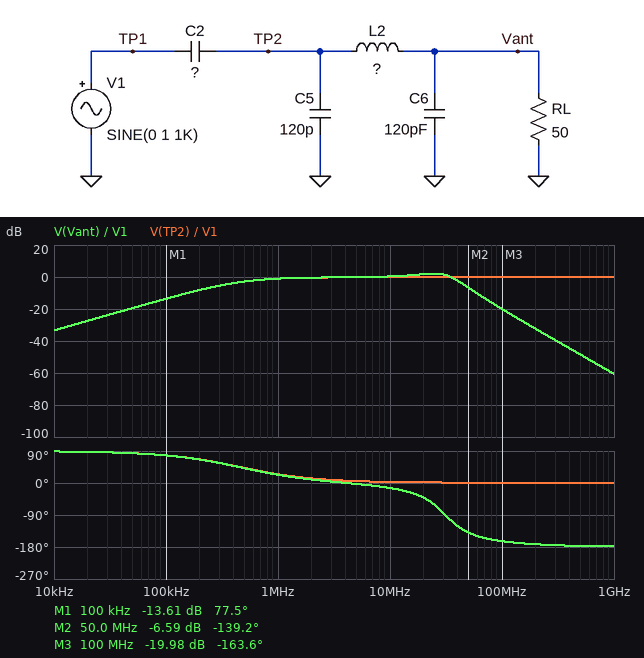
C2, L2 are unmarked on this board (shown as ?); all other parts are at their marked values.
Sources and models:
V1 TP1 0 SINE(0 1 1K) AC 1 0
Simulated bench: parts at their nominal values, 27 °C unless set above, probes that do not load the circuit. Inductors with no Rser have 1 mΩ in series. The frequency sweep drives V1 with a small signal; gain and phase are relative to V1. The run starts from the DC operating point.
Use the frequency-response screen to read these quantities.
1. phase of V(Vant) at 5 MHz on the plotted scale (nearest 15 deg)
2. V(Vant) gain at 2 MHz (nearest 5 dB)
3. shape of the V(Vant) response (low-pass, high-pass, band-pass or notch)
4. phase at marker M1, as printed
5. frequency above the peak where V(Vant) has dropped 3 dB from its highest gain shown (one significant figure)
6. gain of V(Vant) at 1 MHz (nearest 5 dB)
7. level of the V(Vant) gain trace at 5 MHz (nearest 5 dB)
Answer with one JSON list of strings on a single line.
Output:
["0 deg", "0 dB", "band-pass", "77.5 deg", "40 MHz", "0 dB", "0 dB"]
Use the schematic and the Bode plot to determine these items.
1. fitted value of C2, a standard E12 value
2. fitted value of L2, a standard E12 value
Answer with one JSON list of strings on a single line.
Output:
["6.8 nF", "220 nH"]
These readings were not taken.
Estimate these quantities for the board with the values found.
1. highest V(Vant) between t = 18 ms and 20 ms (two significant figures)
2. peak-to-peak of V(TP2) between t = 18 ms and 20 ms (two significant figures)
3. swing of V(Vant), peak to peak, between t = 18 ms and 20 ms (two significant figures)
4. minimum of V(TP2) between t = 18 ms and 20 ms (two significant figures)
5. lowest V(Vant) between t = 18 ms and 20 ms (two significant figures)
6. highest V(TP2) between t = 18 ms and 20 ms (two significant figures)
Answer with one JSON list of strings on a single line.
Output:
["2.1 mV", "4.3 mV", "4.3 mV", "-2.1 mV", "-2.1 mV", "2.1 mV"]
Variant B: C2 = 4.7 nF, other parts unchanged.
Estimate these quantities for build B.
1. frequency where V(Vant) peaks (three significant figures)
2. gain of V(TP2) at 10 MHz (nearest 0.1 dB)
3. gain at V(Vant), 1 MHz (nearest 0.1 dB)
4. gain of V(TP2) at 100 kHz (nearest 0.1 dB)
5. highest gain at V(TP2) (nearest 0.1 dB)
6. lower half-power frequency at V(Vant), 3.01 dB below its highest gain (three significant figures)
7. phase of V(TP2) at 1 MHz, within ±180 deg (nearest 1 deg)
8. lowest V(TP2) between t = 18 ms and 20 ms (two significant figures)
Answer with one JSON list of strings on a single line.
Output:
["25.1 MHz", "-0.3 dB", "-1.8 dB", "-16.7 dB", "0 dB", "1.69 MHz", "33 deg", "-1.5 mV"]
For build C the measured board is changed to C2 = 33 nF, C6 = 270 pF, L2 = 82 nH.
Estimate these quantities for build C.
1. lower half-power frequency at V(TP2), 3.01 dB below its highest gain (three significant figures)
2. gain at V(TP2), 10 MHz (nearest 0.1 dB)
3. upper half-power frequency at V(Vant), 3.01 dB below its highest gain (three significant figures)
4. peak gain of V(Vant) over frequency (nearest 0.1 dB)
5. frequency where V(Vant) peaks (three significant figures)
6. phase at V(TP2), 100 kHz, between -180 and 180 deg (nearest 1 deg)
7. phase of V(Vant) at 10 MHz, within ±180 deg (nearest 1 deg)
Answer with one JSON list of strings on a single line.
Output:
["99.7 kHz", "-0.1 dB", "38.4 MHz", "9.3 dB", "32.9 MHz", "44 deg", "-6 deg"]
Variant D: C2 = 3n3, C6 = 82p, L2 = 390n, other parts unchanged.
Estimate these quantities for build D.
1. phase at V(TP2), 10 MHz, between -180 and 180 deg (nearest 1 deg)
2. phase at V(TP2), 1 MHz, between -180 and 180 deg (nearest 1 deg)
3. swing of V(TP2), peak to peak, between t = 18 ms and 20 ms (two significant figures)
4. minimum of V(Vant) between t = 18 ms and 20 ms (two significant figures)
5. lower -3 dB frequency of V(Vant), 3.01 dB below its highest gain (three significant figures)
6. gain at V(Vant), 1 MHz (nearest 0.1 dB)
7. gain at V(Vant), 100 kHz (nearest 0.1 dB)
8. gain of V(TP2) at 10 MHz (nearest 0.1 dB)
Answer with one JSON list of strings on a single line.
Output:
["5 deg", "44 deg", "2.1 mV", "-1.0 mV", "945 kHz", "-2.9 dB", "-19.7 dB", "-0.1 dB"]
